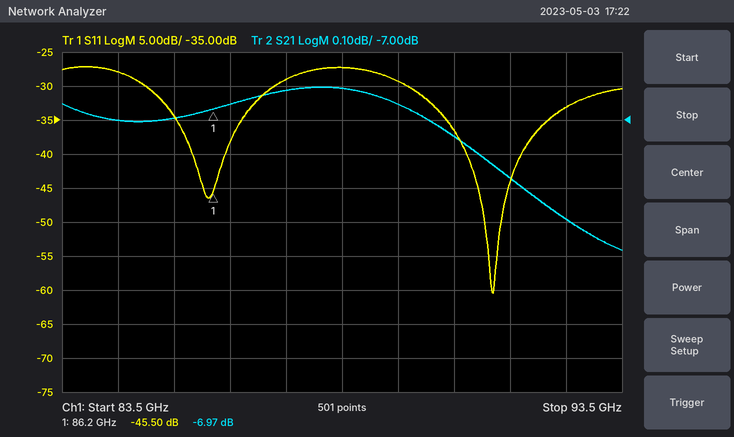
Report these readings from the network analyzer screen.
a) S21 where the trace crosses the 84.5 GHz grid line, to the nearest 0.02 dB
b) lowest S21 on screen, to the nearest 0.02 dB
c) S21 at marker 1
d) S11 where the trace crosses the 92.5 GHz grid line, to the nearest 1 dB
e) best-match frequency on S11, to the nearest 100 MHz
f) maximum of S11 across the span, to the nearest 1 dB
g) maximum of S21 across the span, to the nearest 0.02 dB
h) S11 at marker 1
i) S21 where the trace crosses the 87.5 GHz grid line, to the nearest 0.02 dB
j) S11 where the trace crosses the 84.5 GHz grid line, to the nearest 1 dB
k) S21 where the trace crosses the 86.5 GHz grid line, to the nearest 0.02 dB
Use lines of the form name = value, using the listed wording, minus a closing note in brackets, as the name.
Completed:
S21 where the trace crosses the 84.5 GHz grid line, to the nearest 0.02 dB = -7.00 dB
lowest S21 on screen, to the nearest 0.02 dB = -7.38 dB
S21 at marker 1 = -6.97 dB
S11 where the trace crosses the 92.5 GHz grid line, to the nearest 1 dB = -33 dB
best-match frequency on S11, to the nearest 100 MHz = 91.2 GHz
maximum of S11 across the span, to the nearest 1 dB = -27 dB
maximum of S21 across the span, to the nearest 0.02 dB = -6.90 dB
S11 at marker 1 = -45.50 dB
S21 where the trace crosses the 87.5 GHz grid line, to the nearest 0.02 dB = -6.92 dB
S11 where the trace crosses the 84.5 GHz grid line, to the nearest 1 dB = -28 dB
S21 where the trace crosses the 86.5 GHz grid line, to the nearest 0.02 dB = -6.96 dB
